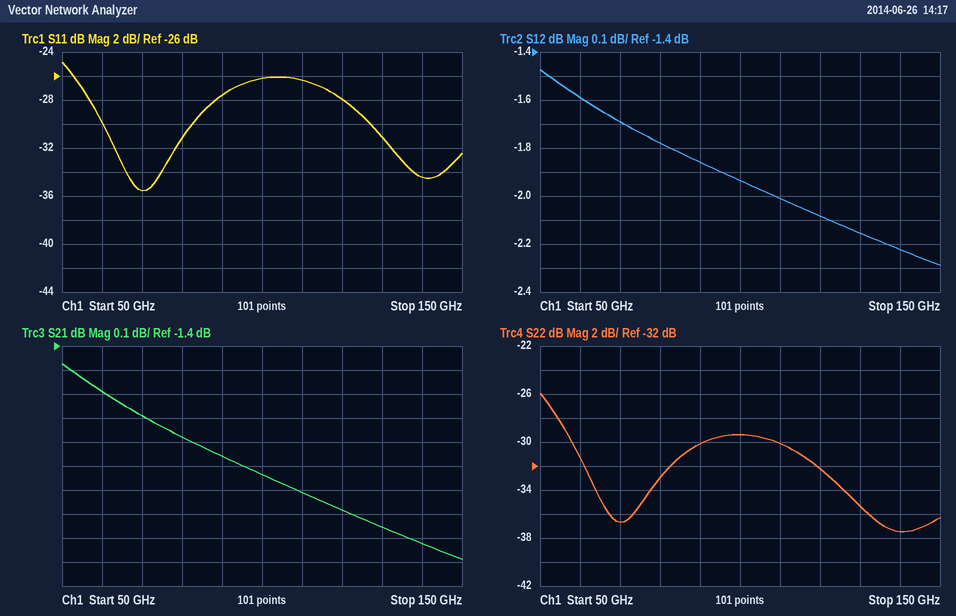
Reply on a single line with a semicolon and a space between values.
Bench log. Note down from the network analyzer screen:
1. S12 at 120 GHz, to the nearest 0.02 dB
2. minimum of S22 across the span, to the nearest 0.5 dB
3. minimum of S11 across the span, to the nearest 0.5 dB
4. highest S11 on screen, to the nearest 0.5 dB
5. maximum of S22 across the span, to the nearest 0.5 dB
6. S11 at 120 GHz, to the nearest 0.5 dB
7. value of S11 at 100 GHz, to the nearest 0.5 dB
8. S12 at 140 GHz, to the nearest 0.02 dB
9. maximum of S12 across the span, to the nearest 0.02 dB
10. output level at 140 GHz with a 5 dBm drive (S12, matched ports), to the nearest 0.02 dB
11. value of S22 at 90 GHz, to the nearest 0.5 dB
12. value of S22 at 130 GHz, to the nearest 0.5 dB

-2.08 dB; -37.5 dB; -35.5 dB; -25.0 dB; -26.0 dB; -28.0 dB; -26.0 dB; -2.22 dB; -1.48 dB; 2.78 dBm; -30.0 dB; -35.5 dB
